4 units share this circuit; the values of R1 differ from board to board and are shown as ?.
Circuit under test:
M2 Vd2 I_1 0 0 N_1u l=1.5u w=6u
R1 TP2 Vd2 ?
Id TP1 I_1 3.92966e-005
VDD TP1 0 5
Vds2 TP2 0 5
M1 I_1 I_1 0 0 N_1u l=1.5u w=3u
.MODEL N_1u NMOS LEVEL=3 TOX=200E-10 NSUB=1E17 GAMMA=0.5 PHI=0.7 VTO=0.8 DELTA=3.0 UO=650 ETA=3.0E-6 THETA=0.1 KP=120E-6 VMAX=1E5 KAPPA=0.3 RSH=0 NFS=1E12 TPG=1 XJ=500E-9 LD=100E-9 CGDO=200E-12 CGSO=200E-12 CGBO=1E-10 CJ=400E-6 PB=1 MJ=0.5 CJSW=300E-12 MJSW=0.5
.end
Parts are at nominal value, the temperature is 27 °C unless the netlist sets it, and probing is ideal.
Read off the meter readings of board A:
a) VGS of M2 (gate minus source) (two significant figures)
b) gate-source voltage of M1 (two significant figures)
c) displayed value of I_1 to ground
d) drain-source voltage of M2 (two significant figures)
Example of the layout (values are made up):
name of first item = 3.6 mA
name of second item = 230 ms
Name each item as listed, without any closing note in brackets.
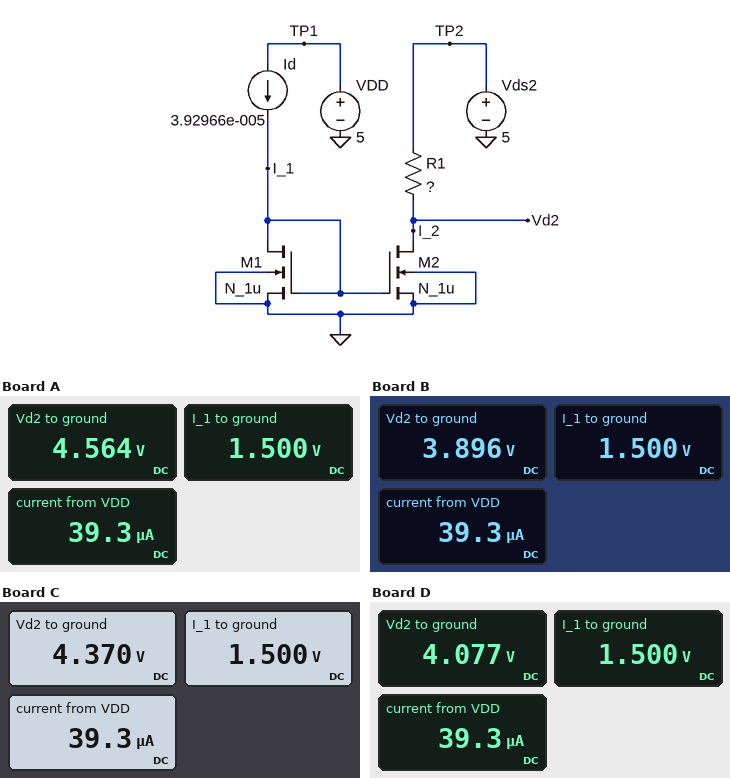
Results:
VGS of M2 (gate minus source) = 1.5 V
gate-source voltage of M1 = 1.5 V
displayed value of I_1 to ground = 1.500 V
drain-source voltage of M2 = 4.6 V
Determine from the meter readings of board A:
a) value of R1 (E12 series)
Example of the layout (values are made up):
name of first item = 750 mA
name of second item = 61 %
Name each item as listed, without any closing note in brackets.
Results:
value of R1 = 4.7 kΩ
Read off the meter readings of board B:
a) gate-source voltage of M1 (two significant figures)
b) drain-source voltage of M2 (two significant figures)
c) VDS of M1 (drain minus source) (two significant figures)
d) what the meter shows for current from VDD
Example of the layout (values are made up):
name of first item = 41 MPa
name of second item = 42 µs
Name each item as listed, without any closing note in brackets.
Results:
gate-source voltage of M1 = 1.5 V
drain-source voltage of M2 = 3.9 V
VDS of M1 (drain minus source) = 1.5 V
what the meter shows for current from VDD = 39.3 µA
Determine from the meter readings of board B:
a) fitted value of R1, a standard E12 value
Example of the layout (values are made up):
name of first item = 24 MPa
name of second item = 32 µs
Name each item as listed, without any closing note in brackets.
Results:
fitted value of R1, a standard E12 value = 12 kΩ
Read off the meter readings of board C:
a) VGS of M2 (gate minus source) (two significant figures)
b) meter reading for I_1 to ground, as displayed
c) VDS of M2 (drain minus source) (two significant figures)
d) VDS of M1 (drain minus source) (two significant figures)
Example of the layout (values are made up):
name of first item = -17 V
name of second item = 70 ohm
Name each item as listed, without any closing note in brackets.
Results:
VGS of M2 (gate minus source) = 1.5 V
meter reading for I_1 to ground, as displayed = 1.500 V
VDS of M2 (drain minus source) = 4.4 V
VDS of M1 (drain minus source) = 1.5 V
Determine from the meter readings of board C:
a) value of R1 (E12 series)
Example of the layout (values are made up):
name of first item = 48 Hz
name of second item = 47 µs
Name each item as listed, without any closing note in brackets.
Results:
value of R1 = 6.8 kΩ
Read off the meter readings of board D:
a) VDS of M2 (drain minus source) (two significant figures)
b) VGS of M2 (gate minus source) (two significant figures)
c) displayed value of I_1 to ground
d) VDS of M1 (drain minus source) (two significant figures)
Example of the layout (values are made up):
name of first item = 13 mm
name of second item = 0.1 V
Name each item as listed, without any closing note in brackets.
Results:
VDS of M2 (drain minus source) = 4.1 V
VGS of M2 (gate minus source) = 1.5 V
displayed value of I_1 to ground = 1.500 V
VDS of M1 (drain minus source) = 1.5 V
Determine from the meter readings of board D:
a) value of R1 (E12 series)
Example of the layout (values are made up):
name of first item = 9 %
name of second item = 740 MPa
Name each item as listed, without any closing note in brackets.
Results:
value of R1 = 10 kΩ
